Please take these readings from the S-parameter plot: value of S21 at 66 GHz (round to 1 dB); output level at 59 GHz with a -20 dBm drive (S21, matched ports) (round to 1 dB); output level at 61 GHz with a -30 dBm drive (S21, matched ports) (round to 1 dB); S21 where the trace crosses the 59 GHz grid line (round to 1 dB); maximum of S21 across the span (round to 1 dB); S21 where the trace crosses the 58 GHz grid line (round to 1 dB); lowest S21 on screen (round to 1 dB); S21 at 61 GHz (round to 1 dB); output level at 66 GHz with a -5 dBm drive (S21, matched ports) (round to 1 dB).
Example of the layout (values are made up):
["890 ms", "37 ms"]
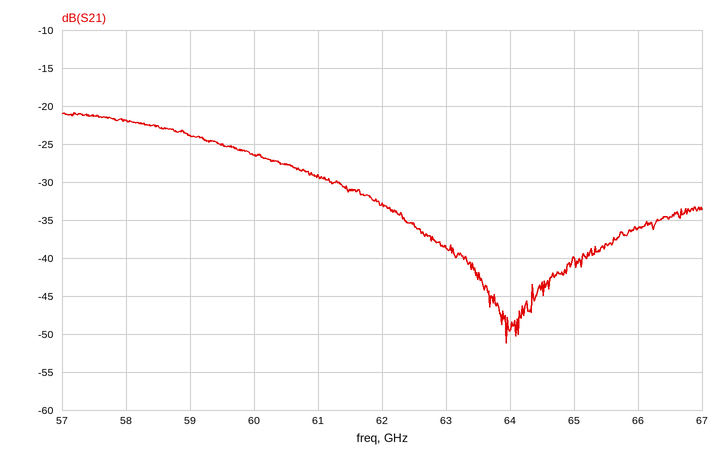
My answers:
["-36 dB", "-44 dBm", "-59 dBm", "-24 dB", "-21 dB", "-22 dB", "-51 dB", "-29 dB", "-41 dBm"]
